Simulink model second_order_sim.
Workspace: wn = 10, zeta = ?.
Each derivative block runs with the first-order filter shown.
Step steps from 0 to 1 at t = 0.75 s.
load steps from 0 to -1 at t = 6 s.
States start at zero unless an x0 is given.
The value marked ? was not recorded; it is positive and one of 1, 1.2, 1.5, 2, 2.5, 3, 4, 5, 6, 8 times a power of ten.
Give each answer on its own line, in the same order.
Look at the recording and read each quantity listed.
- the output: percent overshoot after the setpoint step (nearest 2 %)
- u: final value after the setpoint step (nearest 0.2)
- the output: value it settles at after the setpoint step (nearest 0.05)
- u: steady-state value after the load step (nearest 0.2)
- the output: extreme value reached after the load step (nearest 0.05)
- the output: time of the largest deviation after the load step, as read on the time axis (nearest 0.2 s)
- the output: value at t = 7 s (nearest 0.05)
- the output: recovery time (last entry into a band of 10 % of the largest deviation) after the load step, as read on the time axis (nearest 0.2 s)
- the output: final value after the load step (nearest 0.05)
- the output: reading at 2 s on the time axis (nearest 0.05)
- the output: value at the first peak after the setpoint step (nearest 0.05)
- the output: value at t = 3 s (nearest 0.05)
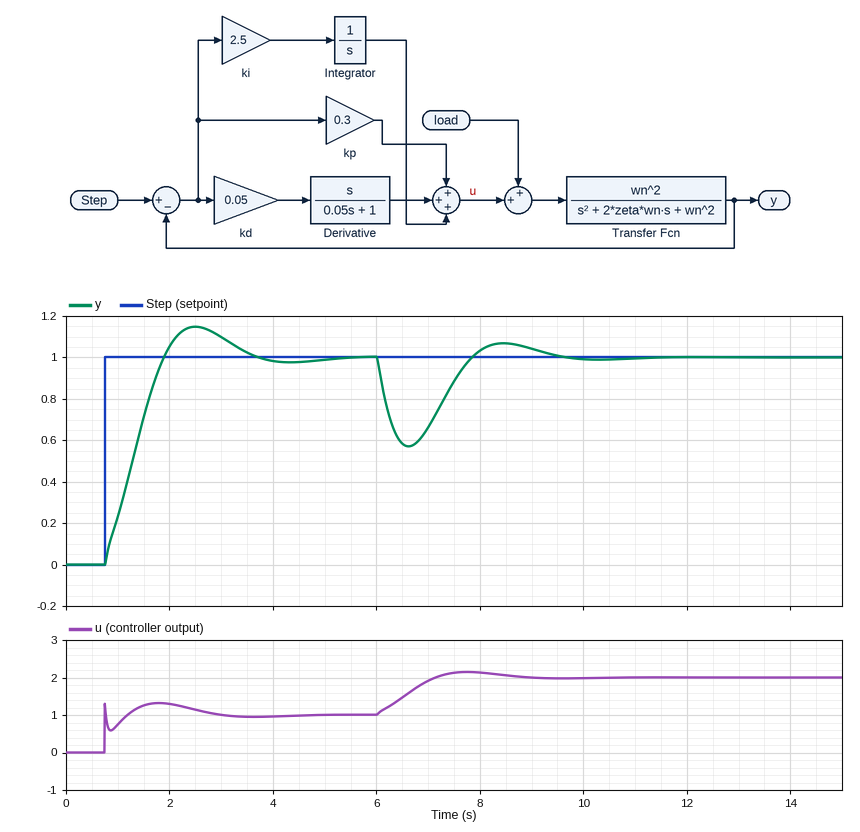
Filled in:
14 %
1.0
1.00
2.0
0.55
6.6 s
0.65
9.0 s
1.00
1.05
1.15
1.10
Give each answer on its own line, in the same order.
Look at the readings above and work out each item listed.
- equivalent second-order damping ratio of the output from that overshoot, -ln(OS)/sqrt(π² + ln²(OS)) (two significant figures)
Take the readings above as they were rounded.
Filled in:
0.53
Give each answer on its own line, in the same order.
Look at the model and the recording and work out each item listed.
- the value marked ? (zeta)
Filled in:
3
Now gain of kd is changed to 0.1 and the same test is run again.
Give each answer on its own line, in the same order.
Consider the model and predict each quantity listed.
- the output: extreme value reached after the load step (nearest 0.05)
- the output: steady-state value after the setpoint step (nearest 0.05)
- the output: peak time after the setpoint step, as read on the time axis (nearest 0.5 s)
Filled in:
0.60
1.00
2.5 s
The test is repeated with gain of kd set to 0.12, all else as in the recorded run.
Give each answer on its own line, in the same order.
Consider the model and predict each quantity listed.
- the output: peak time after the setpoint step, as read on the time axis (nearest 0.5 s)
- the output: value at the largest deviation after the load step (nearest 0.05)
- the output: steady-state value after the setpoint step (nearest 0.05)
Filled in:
2.5 s
0.60
1.00
